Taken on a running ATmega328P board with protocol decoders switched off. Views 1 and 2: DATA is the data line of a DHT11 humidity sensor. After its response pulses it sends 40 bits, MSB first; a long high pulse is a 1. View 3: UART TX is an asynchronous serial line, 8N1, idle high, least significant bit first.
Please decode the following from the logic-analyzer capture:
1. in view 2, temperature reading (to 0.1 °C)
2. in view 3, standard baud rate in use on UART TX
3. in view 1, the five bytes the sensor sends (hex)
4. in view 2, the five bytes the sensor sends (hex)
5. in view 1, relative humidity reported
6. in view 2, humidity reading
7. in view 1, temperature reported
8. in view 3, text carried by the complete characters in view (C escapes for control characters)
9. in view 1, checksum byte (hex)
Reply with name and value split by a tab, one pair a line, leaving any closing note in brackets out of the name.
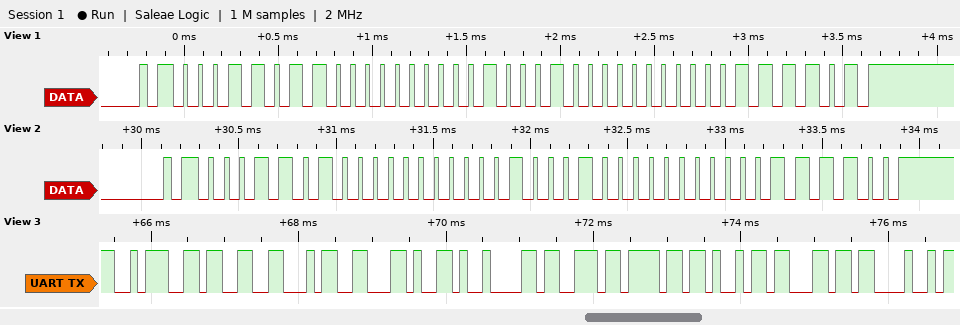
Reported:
in view 2, temperature reading	34.0 °C
in view 3, standard baud rate in use on UART TX	9600 baud
in view 1, the five bytes the sensor sends	1B 00 22 00 3D
in view 2, the five bytes the sensor sends	1A 00 22 00 3C
in view 1, relative humidity reported	27 %
in view 2, humidity reading	26 %
in view 1, temperature reported	34.0 °C
in view 3, text carried by the complete characters in view	":34,\tsoilH"
in view 1, checksum byte	0x3D
